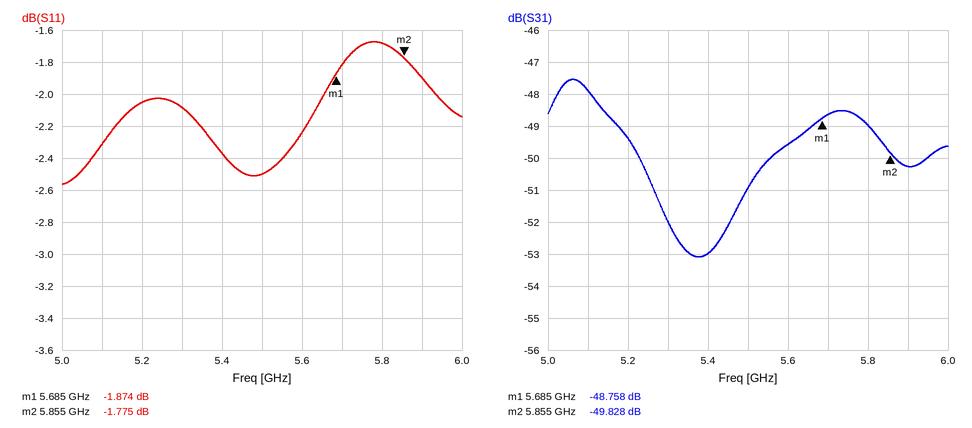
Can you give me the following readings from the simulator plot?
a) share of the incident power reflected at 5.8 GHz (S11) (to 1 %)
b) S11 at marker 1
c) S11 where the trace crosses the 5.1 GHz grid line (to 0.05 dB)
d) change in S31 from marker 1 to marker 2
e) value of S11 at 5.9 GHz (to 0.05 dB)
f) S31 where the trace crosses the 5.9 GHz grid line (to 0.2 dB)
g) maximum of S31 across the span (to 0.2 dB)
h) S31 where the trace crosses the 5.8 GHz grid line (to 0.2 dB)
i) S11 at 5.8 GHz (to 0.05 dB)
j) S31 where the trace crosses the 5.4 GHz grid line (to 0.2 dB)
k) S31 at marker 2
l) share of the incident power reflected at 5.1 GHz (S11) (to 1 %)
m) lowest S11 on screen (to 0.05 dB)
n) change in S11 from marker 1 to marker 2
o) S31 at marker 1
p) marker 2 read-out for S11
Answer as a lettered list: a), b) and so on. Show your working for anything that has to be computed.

a) 10^(-1.7/10) ≈ 68 %
b) -1.874 dB
c) -2.30 dB
d) -49.828 − (-48.758) = -1.070 dB
e) -1.90 dB
f) -50.2 dB
g) -47.6 dB
h) -49.0 dB
i) -1.70 dB
j) -53.0 dB
k) -49.828 dB
l) 10^(-2.3/10) ≈ 59 %
m) -2.55 dB
n) -1.775 − (-1.874) = 0.099 dB
o) -48.758 dB
p) -1.775 dB
